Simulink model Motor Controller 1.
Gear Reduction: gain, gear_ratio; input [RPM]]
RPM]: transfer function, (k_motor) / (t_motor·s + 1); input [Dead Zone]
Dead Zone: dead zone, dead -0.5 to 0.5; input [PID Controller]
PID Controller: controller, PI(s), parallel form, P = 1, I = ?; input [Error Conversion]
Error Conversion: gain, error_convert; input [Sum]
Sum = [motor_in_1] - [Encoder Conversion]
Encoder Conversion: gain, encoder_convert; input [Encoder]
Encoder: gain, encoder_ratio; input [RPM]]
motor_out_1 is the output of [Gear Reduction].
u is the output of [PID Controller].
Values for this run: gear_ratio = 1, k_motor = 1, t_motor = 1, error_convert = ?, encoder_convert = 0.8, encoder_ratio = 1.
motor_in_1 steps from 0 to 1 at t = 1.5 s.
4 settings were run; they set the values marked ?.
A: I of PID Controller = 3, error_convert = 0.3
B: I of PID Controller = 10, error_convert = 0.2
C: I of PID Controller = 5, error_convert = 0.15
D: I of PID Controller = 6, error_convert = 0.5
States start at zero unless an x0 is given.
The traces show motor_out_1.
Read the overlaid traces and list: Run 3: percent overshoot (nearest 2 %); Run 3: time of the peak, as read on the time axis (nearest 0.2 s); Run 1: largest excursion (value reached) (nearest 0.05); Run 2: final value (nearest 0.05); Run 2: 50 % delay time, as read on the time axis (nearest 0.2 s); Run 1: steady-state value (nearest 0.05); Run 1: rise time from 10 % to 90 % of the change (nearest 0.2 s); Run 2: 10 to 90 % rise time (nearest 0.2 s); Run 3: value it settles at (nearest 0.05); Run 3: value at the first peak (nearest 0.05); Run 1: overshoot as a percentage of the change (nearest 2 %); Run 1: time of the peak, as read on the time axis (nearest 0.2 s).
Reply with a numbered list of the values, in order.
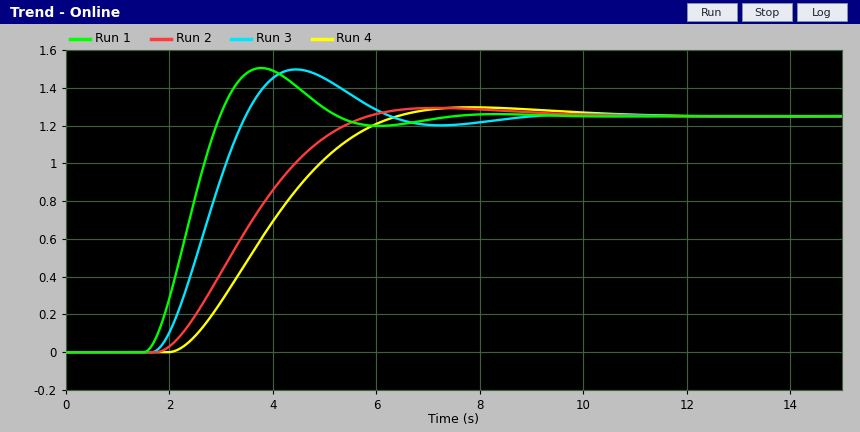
1. 20 %
2. 4.4 s
3. 1.50
4. 1.25
5. 3.4 s
6. 1.25
7. 1.0 s
8. 2.6 s
9. 1.25
10. 1.50
11. 20 %
12. 3.8 s
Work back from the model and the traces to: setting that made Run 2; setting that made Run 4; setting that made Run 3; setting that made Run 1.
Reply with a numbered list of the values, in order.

1. A
2. C
3. B
4. D
